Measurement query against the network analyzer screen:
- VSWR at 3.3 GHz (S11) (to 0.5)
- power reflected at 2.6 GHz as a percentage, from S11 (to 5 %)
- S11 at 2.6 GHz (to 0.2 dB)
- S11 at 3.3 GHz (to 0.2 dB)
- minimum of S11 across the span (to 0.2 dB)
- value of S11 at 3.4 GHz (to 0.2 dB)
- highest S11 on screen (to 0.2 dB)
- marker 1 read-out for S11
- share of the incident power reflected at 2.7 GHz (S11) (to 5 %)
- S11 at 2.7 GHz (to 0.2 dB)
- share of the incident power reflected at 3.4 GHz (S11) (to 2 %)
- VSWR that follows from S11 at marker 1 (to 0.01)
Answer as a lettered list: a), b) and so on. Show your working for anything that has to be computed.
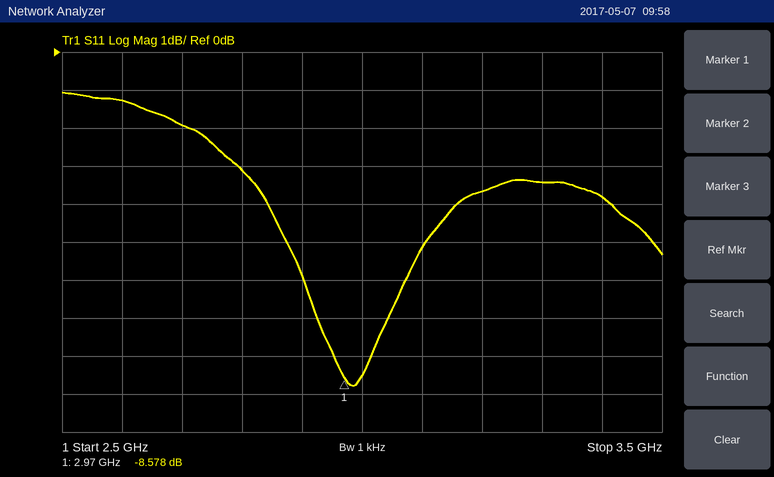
a) |Γ| = 10^(-3.4/20) = 0.6761; VSWR = (1 + 0.6761)/(1 − 0.6761) ≈ 5.17, so 5.0 to the nearest 0.5
b) 10^(-1.2/10) ≈ 75.9 %, so 75 % to the nearest 5 %
c) -1.2 dB
d) -3.4 dB
e) -8.8 dB
f) -3.8 dB
g) -1.0 dB
h) -8.578 dB
i) 10^(-2/10) ≈ 63.1 %, so 65 % to the nearest 5 %
j) -2.0 dB
k) 10^(-3.8/10) ≈ 42 %
l) (1 + 0.3725)/(1 − 0.3725) ≈ 2.19
